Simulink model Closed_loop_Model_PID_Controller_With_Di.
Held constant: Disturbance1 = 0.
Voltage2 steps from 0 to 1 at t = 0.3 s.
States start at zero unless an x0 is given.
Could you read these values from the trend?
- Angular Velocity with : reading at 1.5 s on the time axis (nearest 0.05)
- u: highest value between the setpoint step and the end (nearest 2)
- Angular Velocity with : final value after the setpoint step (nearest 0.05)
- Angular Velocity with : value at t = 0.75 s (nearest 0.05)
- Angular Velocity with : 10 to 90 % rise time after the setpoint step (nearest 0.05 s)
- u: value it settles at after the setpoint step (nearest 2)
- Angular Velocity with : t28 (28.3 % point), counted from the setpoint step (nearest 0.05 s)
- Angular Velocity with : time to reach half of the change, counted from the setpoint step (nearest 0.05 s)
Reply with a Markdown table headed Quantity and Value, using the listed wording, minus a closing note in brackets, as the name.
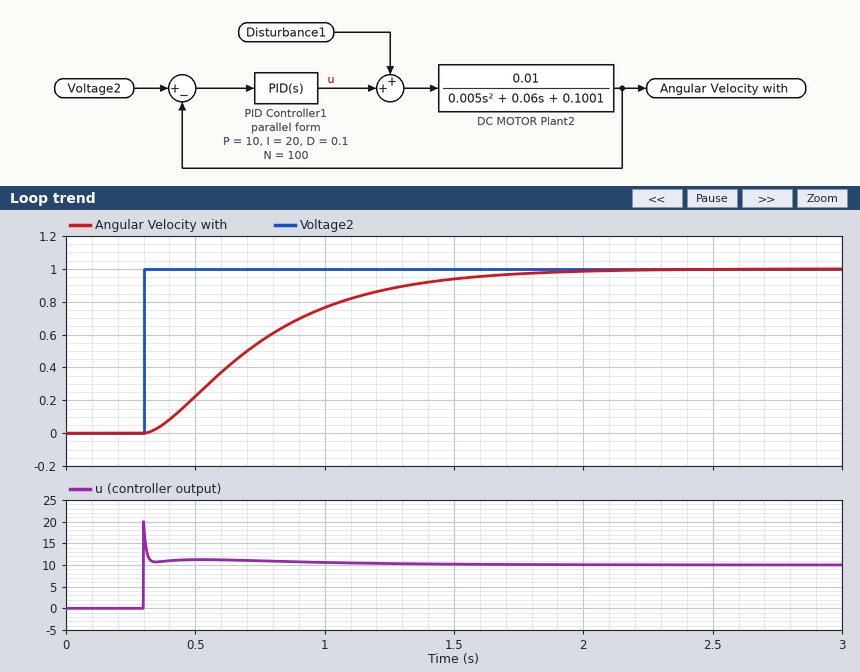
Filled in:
| Quantity | Value |
|---|---|
| Angular Velocity with : reading at 1.5 s on the time axis | 0.95 |
| u: highest value between the setpoint step and the end | 20 |
| Angular Velocity with : final value after the setpoint step | 1.00 |
| Angular Velocity with : value at t = 0.75 s | 0.55 |
| Angular Velocity with : 10 to 90 % rise time after the setpoint step | 0.90 s |
| u: value it settles at after the setpoint step | 10 |
| Angular Velocity with : t28 (28.3 % point), counted from the setpoint step | 0.25 s |
| Angular Velocity with : time to reach half of the change, counted from the setpoint step | 0.40 s |
